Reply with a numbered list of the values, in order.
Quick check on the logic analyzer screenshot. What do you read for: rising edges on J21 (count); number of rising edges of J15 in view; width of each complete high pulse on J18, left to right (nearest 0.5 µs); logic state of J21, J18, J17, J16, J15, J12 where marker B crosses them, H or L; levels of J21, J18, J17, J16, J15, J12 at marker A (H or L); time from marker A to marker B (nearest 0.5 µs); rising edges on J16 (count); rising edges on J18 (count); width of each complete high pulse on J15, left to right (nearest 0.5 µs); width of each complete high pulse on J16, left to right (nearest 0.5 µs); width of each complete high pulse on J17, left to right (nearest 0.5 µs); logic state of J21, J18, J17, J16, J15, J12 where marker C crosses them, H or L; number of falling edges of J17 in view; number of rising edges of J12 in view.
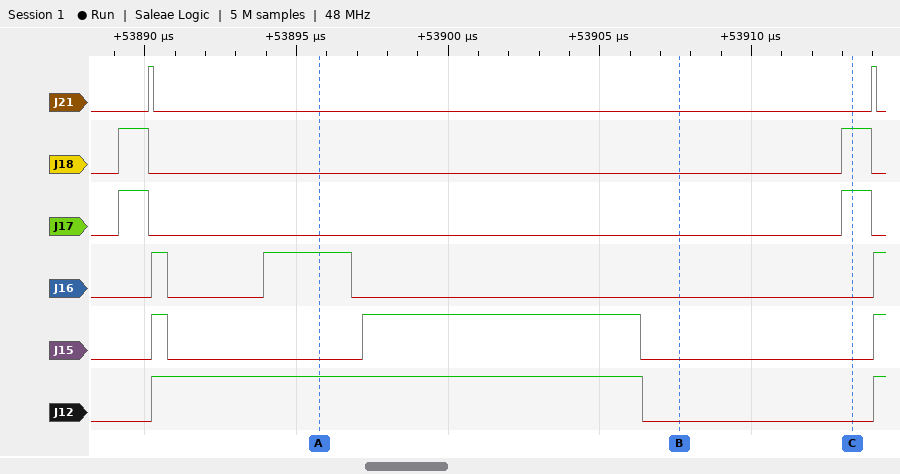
1. 2
2. 3
3. 1 µs, 1 µs
4. J21=L, J18=L, J17=L, J16=L, J15=L, J12=L
5. J21=L, J18=L, J17=L, J16=H, J15=L, J12=H
6. 12 µs
7. 3
8. 2
9. 0.5 µs, 9 µs
10. 0.5 µs, 3 µs
11. 1 µs, 1 µs
12. J21=L, J18=H, J17=H, J16=L, J15=L, J12=L
13. 2
14. 2
